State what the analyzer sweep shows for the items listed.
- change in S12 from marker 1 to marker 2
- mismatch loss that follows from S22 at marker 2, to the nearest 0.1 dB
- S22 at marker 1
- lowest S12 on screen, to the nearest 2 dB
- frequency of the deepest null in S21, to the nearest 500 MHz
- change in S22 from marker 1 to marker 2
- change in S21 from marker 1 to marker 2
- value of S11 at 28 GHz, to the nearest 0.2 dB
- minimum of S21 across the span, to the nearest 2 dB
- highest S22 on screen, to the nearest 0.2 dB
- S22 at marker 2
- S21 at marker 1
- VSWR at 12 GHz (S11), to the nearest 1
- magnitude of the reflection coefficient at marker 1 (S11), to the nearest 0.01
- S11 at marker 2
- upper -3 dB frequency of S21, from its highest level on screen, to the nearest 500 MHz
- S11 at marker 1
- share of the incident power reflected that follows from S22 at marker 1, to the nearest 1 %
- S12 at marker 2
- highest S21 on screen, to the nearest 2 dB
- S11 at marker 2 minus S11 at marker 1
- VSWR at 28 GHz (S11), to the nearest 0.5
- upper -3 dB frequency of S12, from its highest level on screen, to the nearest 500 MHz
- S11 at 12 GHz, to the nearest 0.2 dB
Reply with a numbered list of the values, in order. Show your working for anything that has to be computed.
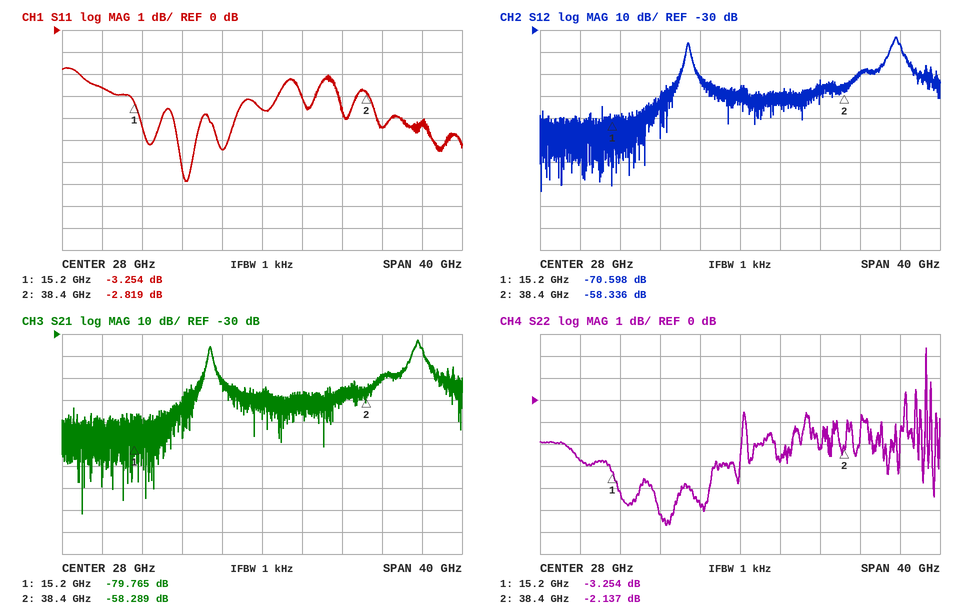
1. -58.336 − (-70.598) = 12.262 dB
2. −10 log10(1 − 10^(-2.137/10)) ≈ 4.1 dB
3. -3.254 dB
4. -104 dB
5. 10.0 GHz
6. -2.137 − (-3.254) = 1.117 dB
7. -58.289 − (-79.765) = 21.476 dB
8. -3.6 dB
9. -112 dB
10. 2.4 dB
11. -2.137 dB
12. -79.765 dB
13. |Γ| = 10^(-2.6/20) = 0.7413; VSWR = (1 + 0.7413)/(1 − 0.7413) ≈ 7
14. 10^(-3.254/20) ≈ 0.69
15. -2.819 dB
16. 44.0 GHz
17. -3.254 dB
18. 10^(-3.254/10) ≈ 47 %
19. -58.336 dB
20. -32 dB
21. -2.819 − (-3.254) = 0.435 dB
22. |Γ| = 10^(-3.6/20) = 0.6607; VSWR = (1 + 0.6607)/(1 − 0.6607) ≈ 4.89, so 5.0 to the nearest 0.5
23. 44.0 GHz
24. -2.6 dB
